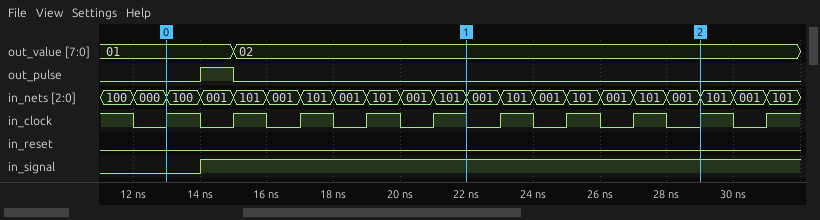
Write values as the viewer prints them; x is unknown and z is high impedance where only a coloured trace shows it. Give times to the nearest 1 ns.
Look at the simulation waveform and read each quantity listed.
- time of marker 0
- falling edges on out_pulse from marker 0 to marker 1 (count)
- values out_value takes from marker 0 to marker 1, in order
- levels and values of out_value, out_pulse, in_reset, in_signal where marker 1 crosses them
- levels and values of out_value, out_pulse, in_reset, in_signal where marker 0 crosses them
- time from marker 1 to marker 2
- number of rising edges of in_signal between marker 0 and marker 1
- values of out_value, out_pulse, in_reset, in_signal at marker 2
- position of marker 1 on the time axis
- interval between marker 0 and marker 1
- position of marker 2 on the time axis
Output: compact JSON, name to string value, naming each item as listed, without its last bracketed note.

{"time of marker 0": "13 ns", "falling edges on out_pulse from marker 0 to marker 1": "1", "values out_value takes from marker 0 to marker 1, in order": "01, 02", "levels and values of out_value, out_pulse, in_reset, in_signal where marker 1 crosses them": "out_value=02, out_pulse=0, in_reset=0, in_signal=1", "levels and values of out_value, out_pulse, in_reset, in_signal where marker 0 crosses them": "out_value=01, out_pulse=0, in_reset=0, in_signal=0", "time from marker 1 to marker 2": "7 ns", "number of rising edges of in_signal between marker 0 and marker 1": "1", "values of out_value, out_pulse, in_reset, in_signal at marker 2": "out_value=02, out_pulse=0, in_reset=0, in_signal=1", "position of marker 1 on the time axis": "22 ns", "interval between marker 0 and marker 1": "9 ns", "position of marker 2 on the time axis": "29 ns"}
